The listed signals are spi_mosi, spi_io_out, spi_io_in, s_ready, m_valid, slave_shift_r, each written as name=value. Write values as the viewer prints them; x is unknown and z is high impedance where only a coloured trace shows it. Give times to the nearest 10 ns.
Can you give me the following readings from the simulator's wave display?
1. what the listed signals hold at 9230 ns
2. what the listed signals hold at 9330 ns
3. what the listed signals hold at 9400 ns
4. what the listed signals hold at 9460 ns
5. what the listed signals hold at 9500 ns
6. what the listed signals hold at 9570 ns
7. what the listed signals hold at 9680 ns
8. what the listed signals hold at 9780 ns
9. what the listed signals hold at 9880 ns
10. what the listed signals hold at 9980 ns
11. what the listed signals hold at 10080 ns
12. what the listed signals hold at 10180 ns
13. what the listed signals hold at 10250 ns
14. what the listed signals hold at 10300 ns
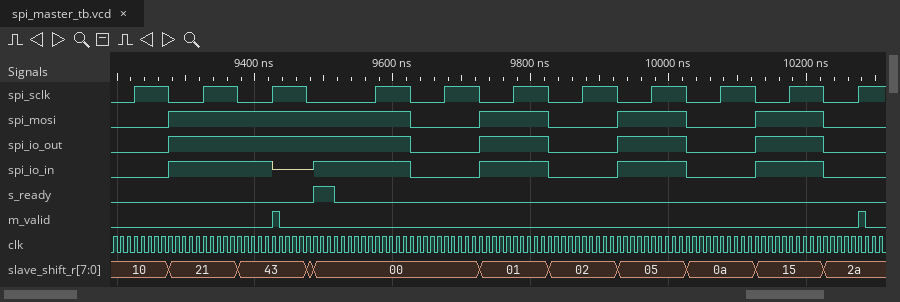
spi_mosi=0, spi_io_out=0, spi_io_in=0, s_ready=0, m_valid=0, slave_shift_r=10
spi_mosi=1, spi_io_out=1, spi_io_in=1, s_ready=0, m_valid=0, slave_shift_r=21
spi_mosi=1, spi_io_out=1, spi_io_in=1, s_ready=0, m_valid=0, slave_shift_r=43
spi_mosi=1, spi_io_out=1, spi_io_in=z, s_ready=0, m_valid=0, slave_shift_r=43
spi_mosi=1, spi_io_out=1, spi_io_in=1, s_ready=1, m_valid=0, slave_shift_r=00
spi_mosi=1, spi_io_out=1, spi_io_in=1, s_ready=0, m_valid=0, slave_shift_r=00
spi_mosi=0, spi_io_out=0, spi_io_in=0, s_ready=0, m_valid=0, slave_shift_r=00
spi_mosi=1, spi_io_out=1, spi_io_in=1, s_ready=0, m_valid=0, slave_shift_r=01
spi_mosi=0, spi_io_out=0, spi_io_in=0, s_ready=0, m_valid=0, slave_shift_r=02
spi_mosi=1, spi_io_out=1, spi_io_in=1, s_ready=0, m_valid=0, slave_shift_r=05
spi_mosi=0, spi_io_out=0, spi_io_in=0, s_ready=0, m_valid=0, slave_shift_r=0a
spi_mosi=1, spi_io_out=1, spi_io_in=1, s_ready=0, m_valid=0, slave_shift_r=15
spi_mosi=0, spi_io_out=0, spi_io_in=0, s_ready=0, m_valid=0, slave_shift_r=2a
spi_mosi=0, spi_io_out=0, spi_io_in=0, s_ready=0, m_valid=0, slave_shift_r=2a
